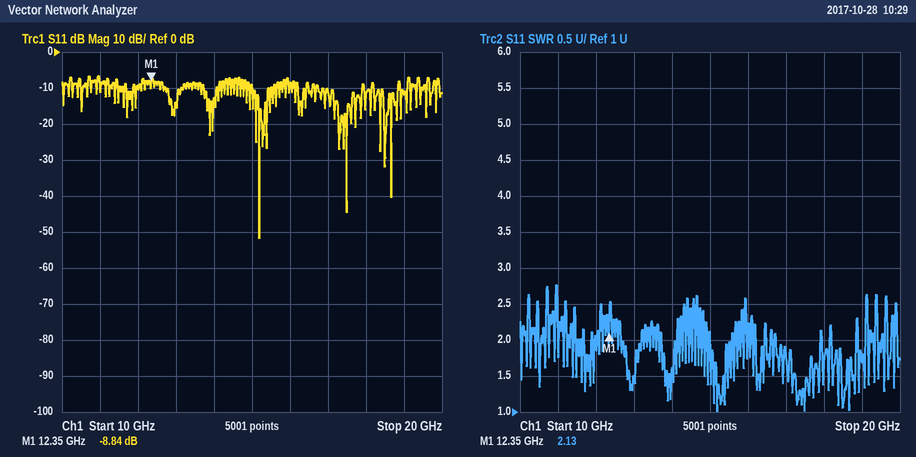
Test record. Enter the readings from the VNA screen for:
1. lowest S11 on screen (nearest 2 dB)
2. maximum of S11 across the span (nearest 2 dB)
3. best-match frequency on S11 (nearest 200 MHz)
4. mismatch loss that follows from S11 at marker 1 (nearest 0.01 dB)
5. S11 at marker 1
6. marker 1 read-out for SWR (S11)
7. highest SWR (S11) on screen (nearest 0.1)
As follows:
-52 dB
-6 dB
15.2 GHz
0.61 dB
-8.84 dB
2.13
2.8
